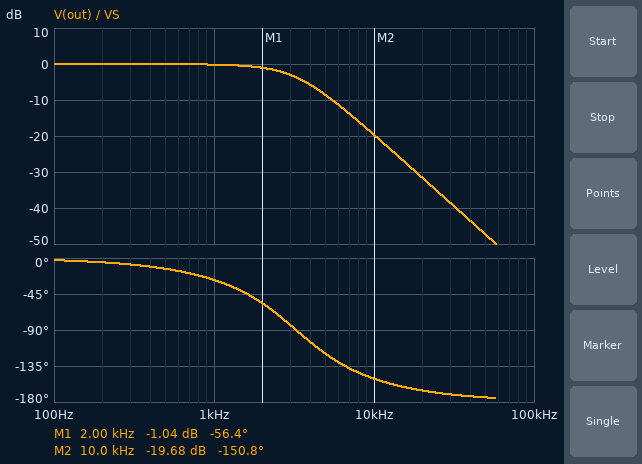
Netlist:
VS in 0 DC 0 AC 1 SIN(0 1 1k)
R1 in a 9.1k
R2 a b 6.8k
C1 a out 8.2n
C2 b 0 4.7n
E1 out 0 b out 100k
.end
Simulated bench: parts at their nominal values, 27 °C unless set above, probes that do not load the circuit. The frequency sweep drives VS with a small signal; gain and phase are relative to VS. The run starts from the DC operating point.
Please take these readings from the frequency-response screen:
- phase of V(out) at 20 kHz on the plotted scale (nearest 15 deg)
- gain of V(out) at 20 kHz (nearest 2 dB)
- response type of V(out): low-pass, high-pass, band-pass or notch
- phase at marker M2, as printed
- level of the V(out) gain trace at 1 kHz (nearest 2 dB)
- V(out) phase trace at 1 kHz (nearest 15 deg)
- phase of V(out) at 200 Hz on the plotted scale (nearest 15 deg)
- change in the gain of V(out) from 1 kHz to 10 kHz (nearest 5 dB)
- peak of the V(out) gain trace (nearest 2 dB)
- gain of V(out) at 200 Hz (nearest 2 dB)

-165 deg
-32 dB
low-pass
-150.8 deg
0 dB
-30 deg
0 deg
-20 dB
0 dB
0 dB
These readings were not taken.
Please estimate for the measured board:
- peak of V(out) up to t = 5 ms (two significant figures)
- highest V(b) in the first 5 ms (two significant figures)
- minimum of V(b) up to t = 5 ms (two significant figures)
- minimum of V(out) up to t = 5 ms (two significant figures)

980 mV
980 mV
-980 mV
-980 mV
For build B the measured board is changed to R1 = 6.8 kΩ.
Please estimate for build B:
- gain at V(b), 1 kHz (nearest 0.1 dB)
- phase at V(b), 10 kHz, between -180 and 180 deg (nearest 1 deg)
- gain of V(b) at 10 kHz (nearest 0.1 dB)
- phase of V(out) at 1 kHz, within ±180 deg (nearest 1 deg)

-0.1 dB
-146 deg
-17.2 dB
-23 deg
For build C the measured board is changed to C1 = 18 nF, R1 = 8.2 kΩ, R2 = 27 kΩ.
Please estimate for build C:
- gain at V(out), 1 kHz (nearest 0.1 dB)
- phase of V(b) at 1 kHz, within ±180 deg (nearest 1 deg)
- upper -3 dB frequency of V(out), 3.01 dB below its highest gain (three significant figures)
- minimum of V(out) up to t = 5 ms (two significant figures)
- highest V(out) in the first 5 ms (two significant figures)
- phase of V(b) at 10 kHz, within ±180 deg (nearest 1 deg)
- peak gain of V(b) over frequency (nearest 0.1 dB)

-0.6 dB
-76 deg
1.29 kHz
-930 mV
930 mV
-172 deg
0.3 dB
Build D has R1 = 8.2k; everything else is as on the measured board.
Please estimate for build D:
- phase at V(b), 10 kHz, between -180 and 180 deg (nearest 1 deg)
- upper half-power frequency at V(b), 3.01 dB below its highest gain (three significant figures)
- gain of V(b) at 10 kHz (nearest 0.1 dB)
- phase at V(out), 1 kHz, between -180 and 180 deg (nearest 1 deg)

-149 deg
3.18 kHz
-18.8 dB
-26 deg
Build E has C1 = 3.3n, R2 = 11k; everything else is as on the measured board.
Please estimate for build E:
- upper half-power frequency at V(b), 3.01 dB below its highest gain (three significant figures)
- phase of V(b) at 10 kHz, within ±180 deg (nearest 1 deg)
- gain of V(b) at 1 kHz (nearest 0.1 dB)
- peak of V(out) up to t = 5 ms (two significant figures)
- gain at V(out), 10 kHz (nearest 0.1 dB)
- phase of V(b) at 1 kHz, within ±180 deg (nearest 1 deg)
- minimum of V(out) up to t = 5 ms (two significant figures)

2.02 kHz
-131 deg
-0.9 dB
910 mV
-17.9 dB
-32 deg
-900 mV
